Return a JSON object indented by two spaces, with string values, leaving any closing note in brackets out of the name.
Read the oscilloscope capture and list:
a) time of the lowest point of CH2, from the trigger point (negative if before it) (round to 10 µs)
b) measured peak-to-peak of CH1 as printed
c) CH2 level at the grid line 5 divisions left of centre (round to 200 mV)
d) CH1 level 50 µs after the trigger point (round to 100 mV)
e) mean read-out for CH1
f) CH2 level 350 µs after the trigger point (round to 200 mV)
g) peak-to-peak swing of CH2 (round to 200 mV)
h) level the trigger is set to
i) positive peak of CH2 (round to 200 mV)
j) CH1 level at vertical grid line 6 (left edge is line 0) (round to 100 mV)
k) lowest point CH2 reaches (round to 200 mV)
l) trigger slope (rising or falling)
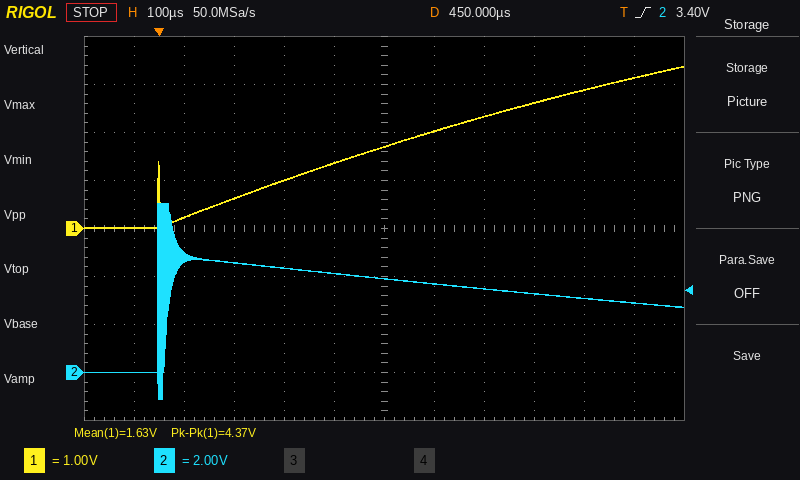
{
  "time of the lowest point of CH2, from the trigger point (negative if before it)": "0 µs",
  "measured peak-to-peak of CH1 as printed": "4.37 V",
  "CH2 level at the grid line 5 divisions left of centre": "0.0 V",
  "CH1 level 50 µs after the trigger point": "200 mV",
  "mean read-out for CH1": "1.63 V",
  "CH2 level 350 µs after the trigger point": "4.2 V",
  "peak-to-peak swing of CH2": "8.2 V",
  "level the trigger is set to": "3.40 V",
  "positive peak of CH2": "7.0 V",
  "CH1 level at vertical grid line 6 (left edge is line 0)": "1.7 V",
  "lowest point CH2 reaches": "-1.2 V",
  "trigger slope": "rising"
}
